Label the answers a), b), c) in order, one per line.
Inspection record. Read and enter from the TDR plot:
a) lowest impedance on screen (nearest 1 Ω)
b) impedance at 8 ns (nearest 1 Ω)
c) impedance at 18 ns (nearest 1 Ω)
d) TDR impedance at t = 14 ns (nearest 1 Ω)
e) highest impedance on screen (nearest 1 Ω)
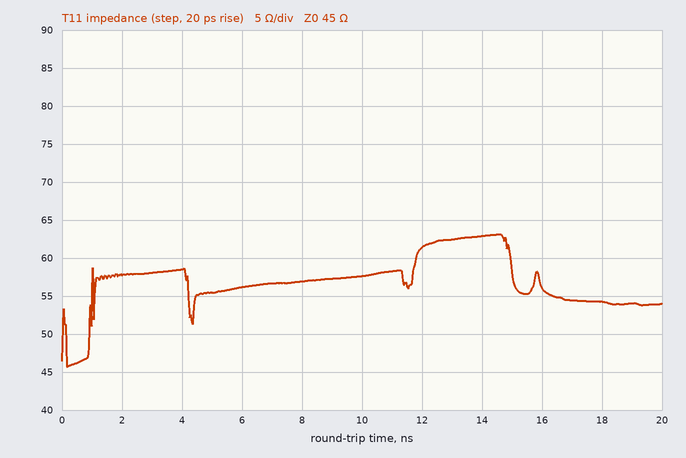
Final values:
a) 46 Ω
b) 57 Ω
c) 54 Ω
d) 63 Ω
e) 63 Ω
